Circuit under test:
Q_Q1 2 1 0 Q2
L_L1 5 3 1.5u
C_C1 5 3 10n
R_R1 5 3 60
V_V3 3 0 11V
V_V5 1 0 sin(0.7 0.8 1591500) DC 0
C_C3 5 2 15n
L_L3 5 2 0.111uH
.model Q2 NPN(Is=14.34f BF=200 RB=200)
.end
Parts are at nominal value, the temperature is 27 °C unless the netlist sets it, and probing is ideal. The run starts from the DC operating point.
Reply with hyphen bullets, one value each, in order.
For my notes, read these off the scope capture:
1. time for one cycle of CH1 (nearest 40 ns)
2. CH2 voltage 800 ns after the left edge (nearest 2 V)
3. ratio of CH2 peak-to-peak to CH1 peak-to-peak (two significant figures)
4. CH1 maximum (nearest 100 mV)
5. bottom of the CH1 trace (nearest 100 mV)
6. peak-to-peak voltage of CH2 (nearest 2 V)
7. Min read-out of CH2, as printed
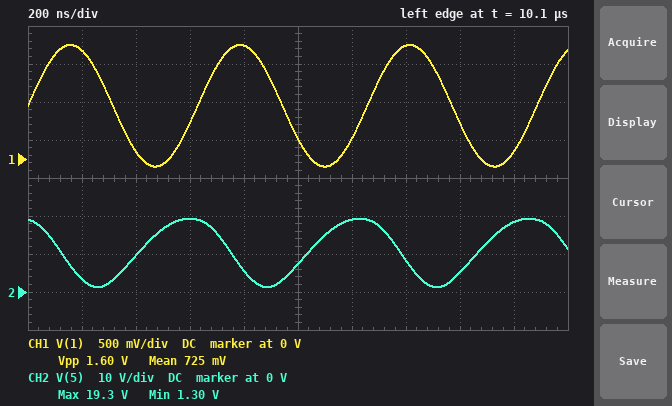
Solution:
- 640 ns
- 6 V
- 11
- 1.5 V
- -100 mV
- 18 V
- 1.30 V
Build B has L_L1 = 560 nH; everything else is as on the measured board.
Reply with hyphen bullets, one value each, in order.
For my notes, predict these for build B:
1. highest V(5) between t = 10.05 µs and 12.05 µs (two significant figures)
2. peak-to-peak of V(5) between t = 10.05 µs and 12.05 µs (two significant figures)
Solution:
- 16 V
- 9.6 V
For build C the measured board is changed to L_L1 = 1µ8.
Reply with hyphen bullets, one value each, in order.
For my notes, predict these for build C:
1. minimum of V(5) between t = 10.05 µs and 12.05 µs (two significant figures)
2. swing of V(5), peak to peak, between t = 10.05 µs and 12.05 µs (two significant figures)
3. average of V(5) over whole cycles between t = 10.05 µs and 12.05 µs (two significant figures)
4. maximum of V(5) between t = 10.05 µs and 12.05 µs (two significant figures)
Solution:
- 3.3 V
- 14 V
- 11 V
- 18 V
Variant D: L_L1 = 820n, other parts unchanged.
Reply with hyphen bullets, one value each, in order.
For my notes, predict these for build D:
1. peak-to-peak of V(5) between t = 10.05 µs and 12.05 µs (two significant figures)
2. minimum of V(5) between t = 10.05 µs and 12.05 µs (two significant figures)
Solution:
- 23 V
- 990 mV
